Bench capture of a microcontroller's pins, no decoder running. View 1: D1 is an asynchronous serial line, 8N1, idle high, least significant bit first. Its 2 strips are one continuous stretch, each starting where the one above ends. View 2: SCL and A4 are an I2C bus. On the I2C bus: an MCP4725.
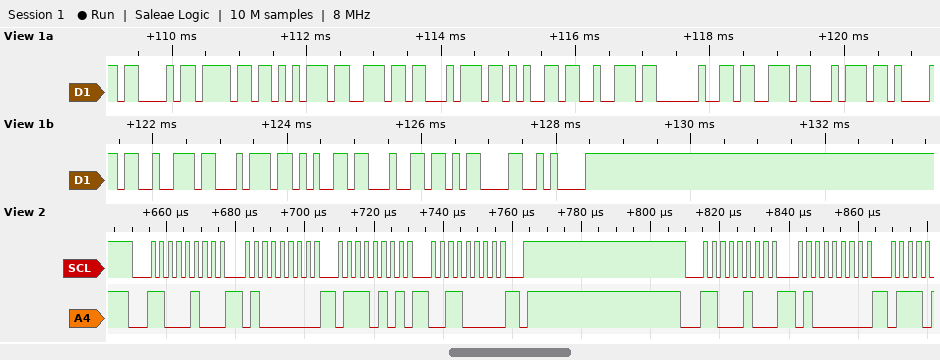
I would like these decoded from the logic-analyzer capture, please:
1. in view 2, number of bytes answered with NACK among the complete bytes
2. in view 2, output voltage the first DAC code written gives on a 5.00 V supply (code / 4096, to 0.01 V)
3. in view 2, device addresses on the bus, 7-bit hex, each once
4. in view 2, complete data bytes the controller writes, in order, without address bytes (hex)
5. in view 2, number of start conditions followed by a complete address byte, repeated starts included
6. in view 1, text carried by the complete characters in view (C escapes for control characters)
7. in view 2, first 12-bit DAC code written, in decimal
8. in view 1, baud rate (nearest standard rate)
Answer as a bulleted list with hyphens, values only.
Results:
- 0
- 2.29 V
- 0x62
- 40 75 30 40
- 2
- "Counter started\r\n"
- 1875
- 9600 baud
